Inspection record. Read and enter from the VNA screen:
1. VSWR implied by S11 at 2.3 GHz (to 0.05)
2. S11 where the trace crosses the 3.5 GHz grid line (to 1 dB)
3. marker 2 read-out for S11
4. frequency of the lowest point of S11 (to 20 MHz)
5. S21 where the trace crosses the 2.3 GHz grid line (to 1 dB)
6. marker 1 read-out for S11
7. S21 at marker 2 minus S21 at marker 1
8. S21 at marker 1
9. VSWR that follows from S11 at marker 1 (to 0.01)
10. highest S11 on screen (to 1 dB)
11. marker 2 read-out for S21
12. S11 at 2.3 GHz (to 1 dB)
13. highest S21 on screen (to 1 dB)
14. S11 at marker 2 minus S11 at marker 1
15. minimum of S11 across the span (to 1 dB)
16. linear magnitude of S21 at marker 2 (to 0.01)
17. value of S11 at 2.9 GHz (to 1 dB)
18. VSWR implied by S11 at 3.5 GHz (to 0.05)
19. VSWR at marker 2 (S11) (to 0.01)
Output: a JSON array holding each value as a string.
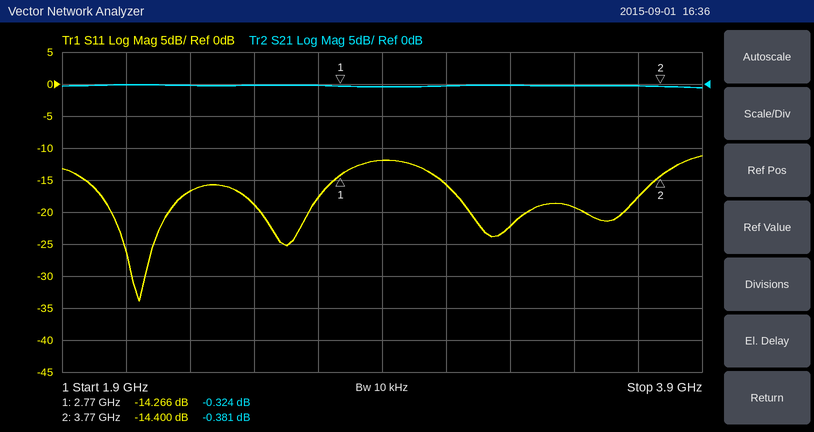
["1.35", "-19 dB", "-14.400 dB", "2.14 GHz", "0 dB", "-14.266 dB", "-0.057 dB", "-0.324 dB", "1.48", "-11 dB", "-0.381 dB", "-17 dB", "0 dB", "-0.134 dB", "-34 dB", "0.96", "-12 dB", "1.25", "1.47"]
